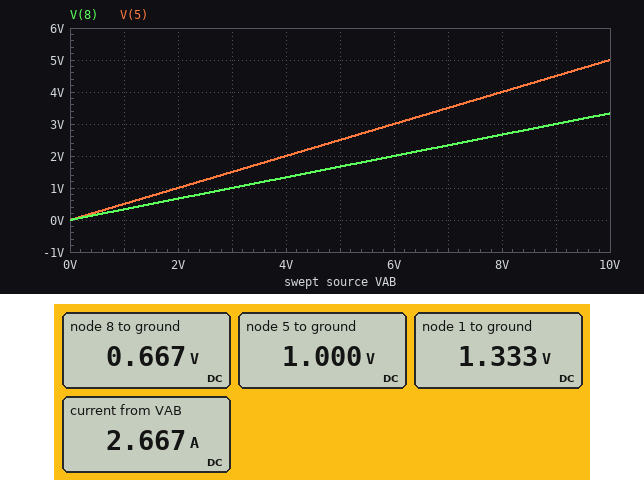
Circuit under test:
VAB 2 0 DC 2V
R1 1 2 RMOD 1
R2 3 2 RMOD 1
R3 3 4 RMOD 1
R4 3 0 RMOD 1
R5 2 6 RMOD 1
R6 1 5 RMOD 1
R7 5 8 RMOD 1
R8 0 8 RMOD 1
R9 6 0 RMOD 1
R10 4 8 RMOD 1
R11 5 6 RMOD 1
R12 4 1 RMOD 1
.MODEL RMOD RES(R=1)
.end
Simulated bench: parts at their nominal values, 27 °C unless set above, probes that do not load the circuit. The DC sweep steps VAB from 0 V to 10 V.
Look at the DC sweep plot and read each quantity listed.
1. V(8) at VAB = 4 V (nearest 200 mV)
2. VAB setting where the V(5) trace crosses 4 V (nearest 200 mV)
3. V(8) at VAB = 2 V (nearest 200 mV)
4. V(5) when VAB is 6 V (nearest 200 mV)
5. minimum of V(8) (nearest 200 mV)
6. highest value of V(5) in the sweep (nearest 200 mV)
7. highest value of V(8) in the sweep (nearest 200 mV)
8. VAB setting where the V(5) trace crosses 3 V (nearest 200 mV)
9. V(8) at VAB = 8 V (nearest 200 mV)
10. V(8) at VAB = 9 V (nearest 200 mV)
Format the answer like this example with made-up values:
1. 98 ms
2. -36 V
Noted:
1. 1.4 V
2. 8.0 V
3. 600 mV
4. 3.0 V
5. 0 V
6. 5.0 V
7. 3.4 V
8. 6.0 V
9. 2.6 V
10. 3.0 V
